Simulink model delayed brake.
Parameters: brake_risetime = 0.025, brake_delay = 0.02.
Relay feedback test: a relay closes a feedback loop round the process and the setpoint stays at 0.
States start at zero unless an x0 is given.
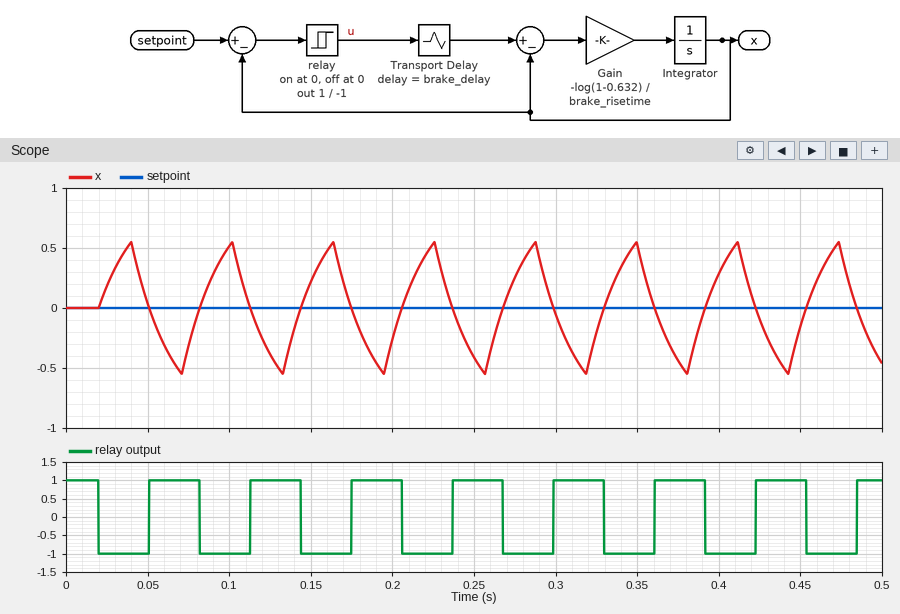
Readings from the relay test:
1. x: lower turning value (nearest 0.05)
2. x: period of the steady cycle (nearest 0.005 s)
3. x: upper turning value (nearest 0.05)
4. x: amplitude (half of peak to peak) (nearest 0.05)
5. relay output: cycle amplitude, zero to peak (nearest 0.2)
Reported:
-0.55
0.060 s
0.55
0.55
1.0
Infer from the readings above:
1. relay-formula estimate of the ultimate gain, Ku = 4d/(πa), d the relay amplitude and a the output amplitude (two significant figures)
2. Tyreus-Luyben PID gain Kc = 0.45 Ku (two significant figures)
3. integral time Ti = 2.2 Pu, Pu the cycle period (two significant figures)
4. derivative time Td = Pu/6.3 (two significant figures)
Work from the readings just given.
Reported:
2.3
1.0
0.13 s
0.0095 s
